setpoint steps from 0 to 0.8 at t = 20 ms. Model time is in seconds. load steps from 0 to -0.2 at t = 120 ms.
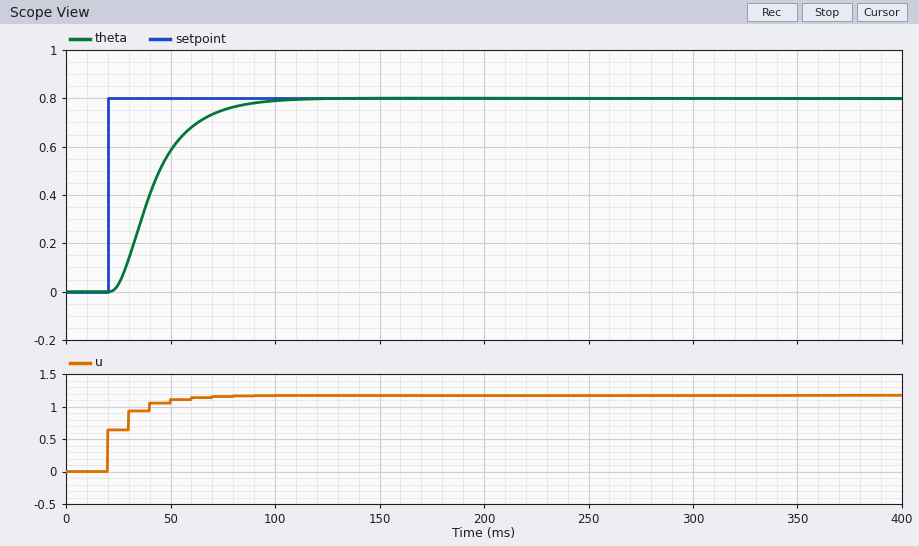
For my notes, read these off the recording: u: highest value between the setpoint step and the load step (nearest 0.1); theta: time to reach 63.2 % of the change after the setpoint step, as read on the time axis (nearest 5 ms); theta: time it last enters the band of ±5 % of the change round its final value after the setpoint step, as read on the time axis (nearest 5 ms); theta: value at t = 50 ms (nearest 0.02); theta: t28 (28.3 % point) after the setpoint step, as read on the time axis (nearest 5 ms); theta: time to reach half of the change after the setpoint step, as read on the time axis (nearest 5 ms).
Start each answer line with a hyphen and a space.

- 1.2
- 45 ms
- 75 ms
- 0.58
- 35 ms
- 40 ms
